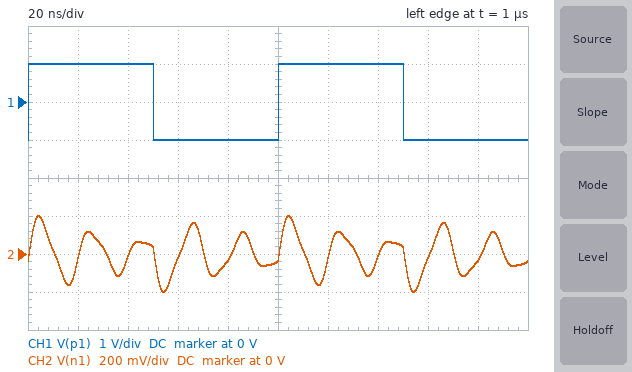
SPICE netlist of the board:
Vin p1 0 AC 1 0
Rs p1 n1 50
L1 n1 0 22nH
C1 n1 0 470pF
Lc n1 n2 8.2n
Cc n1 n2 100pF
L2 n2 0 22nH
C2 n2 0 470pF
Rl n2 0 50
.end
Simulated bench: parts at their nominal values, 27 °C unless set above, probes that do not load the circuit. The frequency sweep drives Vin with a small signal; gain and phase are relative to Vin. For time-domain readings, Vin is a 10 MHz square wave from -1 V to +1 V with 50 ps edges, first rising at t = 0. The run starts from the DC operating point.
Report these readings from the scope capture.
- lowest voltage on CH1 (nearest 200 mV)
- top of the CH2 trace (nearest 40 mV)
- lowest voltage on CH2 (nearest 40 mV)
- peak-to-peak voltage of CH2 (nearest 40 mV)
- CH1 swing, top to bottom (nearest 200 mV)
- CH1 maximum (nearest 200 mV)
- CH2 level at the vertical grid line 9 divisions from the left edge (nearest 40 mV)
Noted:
-1.0 V
200 mV
-200 mV
400 mV
2.0 V
1.0 V
-40 mV
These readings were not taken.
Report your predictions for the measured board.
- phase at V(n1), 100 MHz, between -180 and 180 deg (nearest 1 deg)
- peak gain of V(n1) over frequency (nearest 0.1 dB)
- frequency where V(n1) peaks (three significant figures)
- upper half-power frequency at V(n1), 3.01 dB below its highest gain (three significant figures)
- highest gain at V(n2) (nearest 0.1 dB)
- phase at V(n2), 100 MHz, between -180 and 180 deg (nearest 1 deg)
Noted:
56 deg
-5.9 dB
105 MHz
107 MHz
-6.0 dB
-112 deg
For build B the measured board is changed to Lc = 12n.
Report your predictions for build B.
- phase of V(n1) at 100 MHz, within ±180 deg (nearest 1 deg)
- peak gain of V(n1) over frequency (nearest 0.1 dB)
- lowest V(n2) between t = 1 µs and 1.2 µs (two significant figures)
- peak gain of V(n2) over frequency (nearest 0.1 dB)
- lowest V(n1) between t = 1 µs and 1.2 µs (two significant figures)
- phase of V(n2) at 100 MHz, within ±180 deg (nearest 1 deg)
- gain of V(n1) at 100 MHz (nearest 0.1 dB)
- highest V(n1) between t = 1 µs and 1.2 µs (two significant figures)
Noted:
-79 deg
-5.8 dB
-220 mV
-6.0 dB
-250 mV
109 deg
-15.9 dB
250 mV
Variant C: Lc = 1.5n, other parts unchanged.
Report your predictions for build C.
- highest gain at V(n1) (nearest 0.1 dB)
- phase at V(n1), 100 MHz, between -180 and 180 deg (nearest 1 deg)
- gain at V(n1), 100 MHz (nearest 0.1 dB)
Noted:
-6.0 dB
-84 deg
-28.2 dB
